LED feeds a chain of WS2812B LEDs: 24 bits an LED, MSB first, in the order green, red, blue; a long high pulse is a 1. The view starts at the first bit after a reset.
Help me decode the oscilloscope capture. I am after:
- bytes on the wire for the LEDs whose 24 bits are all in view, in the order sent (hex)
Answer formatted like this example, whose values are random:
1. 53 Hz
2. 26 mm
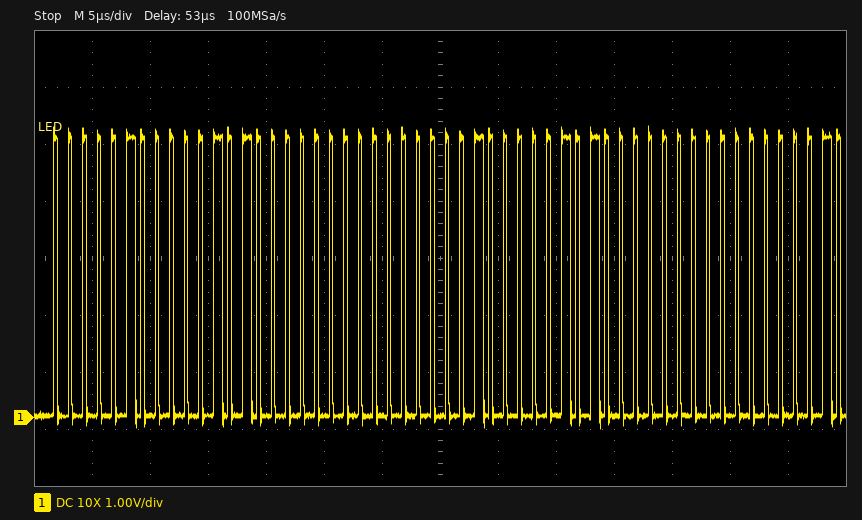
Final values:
1. 04 14 00 04 14 00
